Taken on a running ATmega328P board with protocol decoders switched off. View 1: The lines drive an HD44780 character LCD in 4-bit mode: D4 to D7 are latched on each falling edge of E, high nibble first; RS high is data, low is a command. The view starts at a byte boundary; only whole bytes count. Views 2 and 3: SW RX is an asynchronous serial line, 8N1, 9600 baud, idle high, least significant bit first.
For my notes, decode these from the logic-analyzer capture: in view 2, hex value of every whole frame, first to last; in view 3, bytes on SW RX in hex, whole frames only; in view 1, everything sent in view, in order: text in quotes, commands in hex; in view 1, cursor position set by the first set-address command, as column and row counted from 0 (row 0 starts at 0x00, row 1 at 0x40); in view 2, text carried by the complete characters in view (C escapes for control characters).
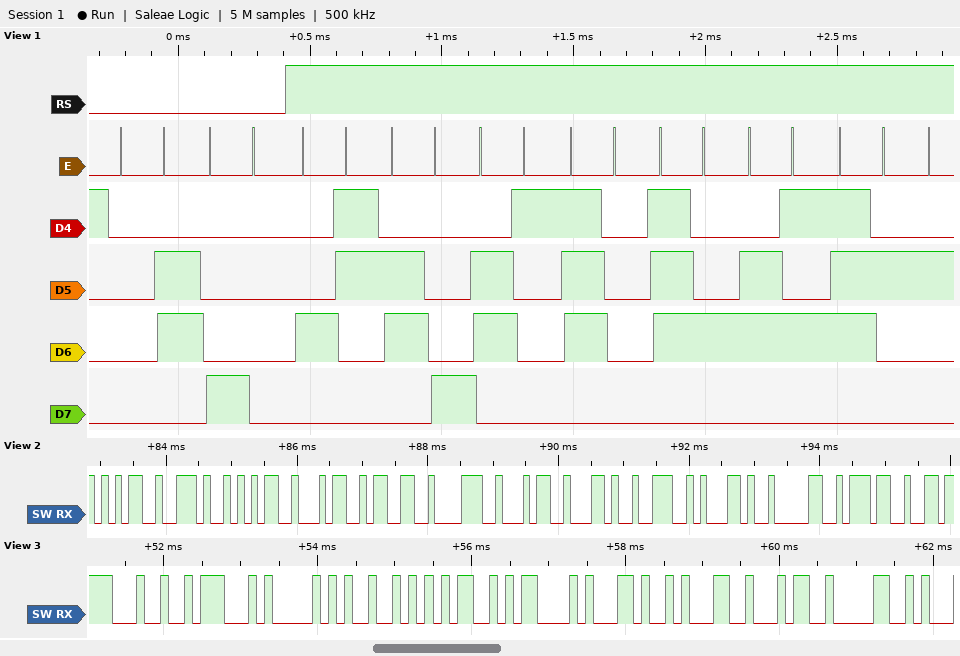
35 2E 35 34 33 38 34 2C 4E 2C 30 37
24 47 50 52 4D 43 2C 31 34 30
0x06 0x80 "Chapter"
column 0, row 0
"5.54384,N,07"
